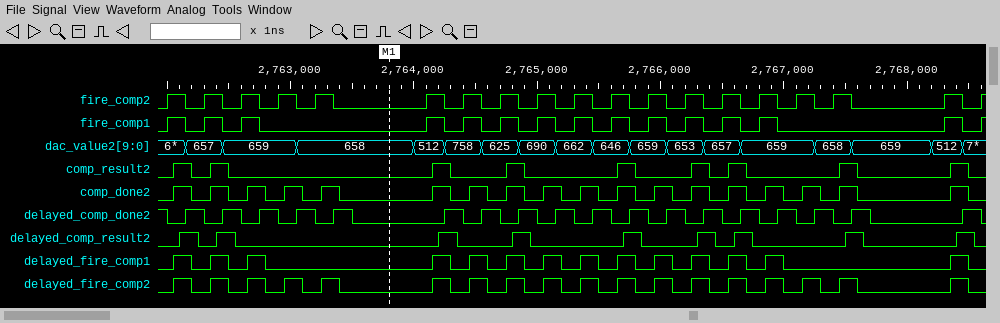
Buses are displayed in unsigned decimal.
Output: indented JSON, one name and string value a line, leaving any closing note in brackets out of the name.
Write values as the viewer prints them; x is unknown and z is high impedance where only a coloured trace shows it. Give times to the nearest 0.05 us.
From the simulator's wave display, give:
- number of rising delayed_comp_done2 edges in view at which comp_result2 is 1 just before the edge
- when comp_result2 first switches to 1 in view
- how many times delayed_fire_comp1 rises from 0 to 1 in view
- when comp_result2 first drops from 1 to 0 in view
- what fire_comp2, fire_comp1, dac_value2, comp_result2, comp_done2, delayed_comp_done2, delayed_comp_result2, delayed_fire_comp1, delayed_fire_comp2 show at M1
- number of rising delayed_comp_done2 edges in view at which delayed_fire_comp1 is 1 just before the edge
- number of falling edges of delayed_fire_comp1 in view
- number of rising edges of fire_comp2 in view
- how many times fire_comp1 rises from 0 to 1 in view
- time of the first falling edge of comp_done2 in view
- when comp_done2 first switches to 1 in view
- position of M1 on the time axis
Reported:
{
  "number of rising delayed_comp_done2 edges in view at which comp_result2 is 1 just before the edge": "9",
  "when comp_result2 first switches to 1 in view": "2762.05 us",
  "how many times delayed_fire_comp1 rises from 0 to 1 in view": "14",
  "when comp_result2 first drops from 1 to 0 in view": "2762.2 us",
  "what fire_comp2, fire_comp1, dac_value2, comp_result2, comp_done2, delayed_comp_done2, delayed_comp_result2, delayed_fire_comp1, delayed_fire_comp2 show at M1": "fire_comp2=0, fire_comp1=0, dac_value2=658, comp_result2=0, comp_done2=0, delayed_comp_done2=0, delayed_comp_result2=0, delayed_fire_comp1=0, delayed_fire_comp2=0",
  "number of rising delayed_comp_done2 edges in view at which delayed_fire_comp1 is 1 just before the edge": "14",
  "number of falling edges of delayed_fire_comp1 in view": "14",
  "number of rising edges of fire_comp2 in view": "19",
  "how many times fire_comp1 rises from 0 to 1 in view": "15",
  "time of the first falling edge of comp_done2 in view": "2762.2 us",
  "when comp_done2 first switches to 1 in view": "2762.05 us",
  "position of M1 on the time axis": "2763.8 us"
}
